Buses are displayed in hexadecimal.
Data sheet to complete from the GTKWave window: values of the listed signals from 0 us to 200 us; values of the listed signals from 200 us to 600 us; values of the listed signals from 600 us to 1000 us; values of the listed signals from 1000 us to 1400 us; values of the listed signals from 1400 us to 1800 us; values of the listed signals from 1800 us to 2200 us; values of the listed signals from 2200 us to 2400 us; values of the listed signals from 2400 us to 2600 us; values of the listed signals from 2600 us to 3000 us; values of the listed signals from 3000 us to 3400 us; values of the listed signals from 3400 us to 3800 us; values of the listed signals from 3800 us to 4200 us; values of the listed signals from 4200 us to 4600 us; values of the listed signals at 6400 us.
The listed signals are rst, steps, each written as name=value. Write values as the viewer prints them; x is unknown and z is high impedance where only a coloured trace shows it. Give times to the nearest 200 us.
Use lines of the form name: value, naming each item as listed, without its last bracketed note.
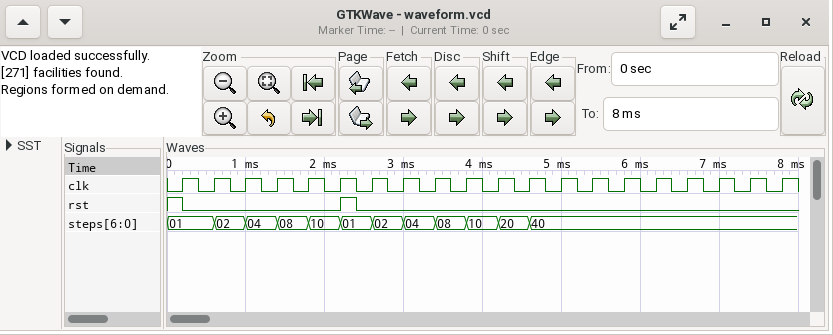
values of the listed signals from 0 us to 200 us: rst=1, steps=01
values of the listed signals from 200 us to 600 us: rst=0, steps=01
values of the listed signals from 600 us to 1000 us: rst=0, steps=02
values of the listed signals from 1000 us to 1400 us: rst=0, steps=04
values of the listed signals from 1400 us to 1800 us: rst=0, steps=08
values of the listed signals from 1800 us to 2200 us: rst=0, steps=10
values of the listed signals from 2200 us to 2400 us: rst=1, steps=01
values of the listed signals from 2400 us to 2600 us: rst=0, steps=01
values of the listed signals from 2600 us to 3000 us: rst=0, steps=02
values of the listed signals from 3000 us to 3400 us: rst=0, steps=04
values of the listed signals from 3400 us to 3800 us: rst=0, steps=08
values of the listed signals from 3800 us to 4200 us: rst=0, steps=10
values of the listed signals from 4200 us to 4600 us: rst=0, steps=20
values of the listed signals at 6400 us: rst=0, steps=40
